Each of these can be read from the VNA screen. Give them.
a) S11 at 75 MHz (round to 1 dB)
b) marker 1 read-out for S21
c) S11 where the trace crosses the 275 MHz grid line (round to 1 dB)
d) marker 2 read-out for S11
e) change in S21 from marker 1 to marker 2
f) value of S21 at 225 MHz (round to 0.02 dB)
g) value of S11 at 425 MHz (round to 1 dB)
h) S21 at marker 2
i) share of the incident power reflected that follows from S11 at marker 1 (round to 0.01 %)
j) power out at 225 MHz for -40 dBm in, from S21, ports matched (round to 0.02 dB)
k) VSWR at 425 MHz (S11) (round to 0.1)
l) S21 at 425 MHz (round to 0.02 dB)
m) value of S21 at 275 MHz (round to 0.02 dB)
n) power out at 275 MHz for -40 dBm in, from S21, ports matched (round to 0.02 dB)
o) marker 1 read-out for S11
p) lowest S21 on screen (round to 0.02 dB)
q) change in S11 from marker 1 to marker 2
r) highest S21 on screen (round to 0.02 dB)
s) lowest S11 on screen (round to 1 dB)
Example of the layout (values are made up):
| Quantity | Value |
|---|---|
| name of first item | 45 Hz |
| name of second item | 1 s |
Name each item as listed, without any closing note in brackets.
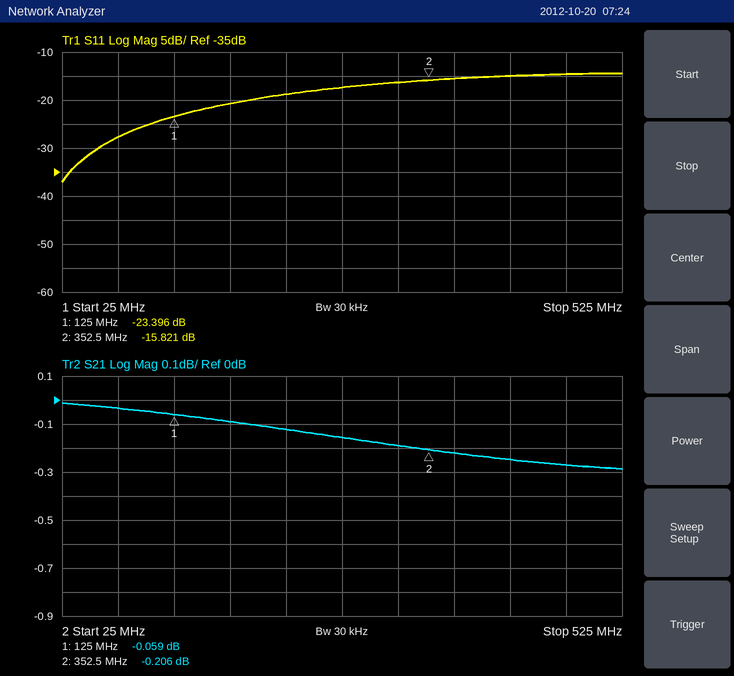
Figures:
| Quantity | Value |
|---|---|
| S11 at 75 MHz | -28 dB |
| marker 1 read-out for S21 | -0.059 dB |
| S11 where the trace crosses the 275 MHz grid line | -17 dB |
| marker 2 read-out for S11 | -15.821 dB |
| change in S21 from marker 1 to marker 2 | -0.147 dB |
| value of S21 at 225 MHz | -0.12 dB |
| value of S11 at 425 MHz | -15 dB |
| S21 at marker 2 | -0.206 dB |
| share of the incident power reflected that follows from S11 at marker 1 | 0.46 % |
| power out at 225 MHz for -40 dBm in, from S21, ports matched | -40.12 dBm |
| VSWR at 425 MHz (S11) | 1.4 |
| S21 at 425 MHz | -0.24 dB |
| value of S21 at 275 MHz | -0.16 dB |
| power out at 275 MHz for -40 dBm in, from S21, ports matched | -40.16 dBm |
| marker 1 read-out for S11 | -23.396 dB |
| lowest S21 on screen | -0.28 dB |
| change in S11 from marker 1 to marker 2 | 7.575 dB |
| highest S21 on screen | -0.02 dB |
| lowest S11 on screen | -37 dB |
